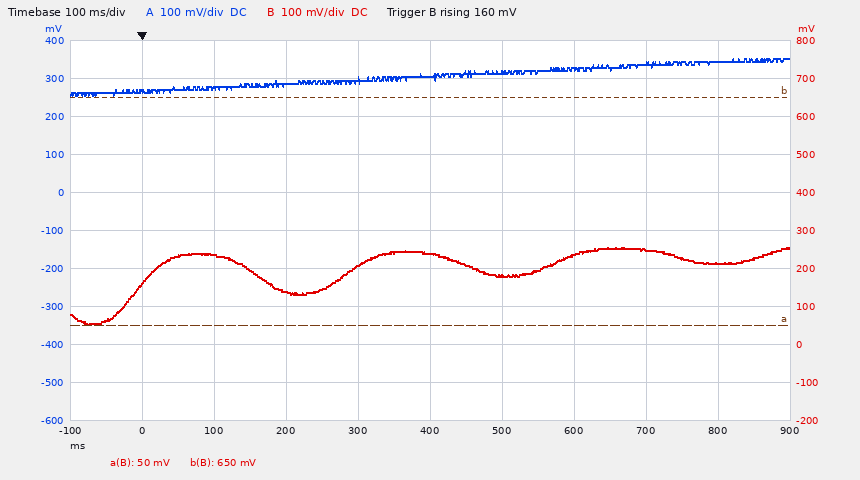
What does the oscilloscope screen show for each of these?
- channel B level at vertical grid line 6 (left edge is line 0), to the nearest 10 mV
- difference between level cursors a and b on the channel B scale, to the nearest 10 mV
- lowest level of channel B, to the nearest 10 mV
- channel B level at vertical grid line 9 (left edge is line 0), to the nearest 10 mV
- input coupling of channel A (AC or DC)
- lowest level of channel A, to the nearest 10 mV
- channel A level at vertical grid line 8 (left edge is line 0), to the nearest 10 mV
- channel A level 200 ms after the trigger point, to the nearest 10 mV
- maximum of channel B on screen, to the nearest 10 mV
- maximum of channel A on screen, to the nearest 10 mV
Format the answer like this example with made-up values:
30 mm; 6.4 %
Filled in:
180 mV; 600 mV; 50 mV; 210 mV; DC; 260 mV; 340 mV; 280 mV; 260 mV; 350 mV
